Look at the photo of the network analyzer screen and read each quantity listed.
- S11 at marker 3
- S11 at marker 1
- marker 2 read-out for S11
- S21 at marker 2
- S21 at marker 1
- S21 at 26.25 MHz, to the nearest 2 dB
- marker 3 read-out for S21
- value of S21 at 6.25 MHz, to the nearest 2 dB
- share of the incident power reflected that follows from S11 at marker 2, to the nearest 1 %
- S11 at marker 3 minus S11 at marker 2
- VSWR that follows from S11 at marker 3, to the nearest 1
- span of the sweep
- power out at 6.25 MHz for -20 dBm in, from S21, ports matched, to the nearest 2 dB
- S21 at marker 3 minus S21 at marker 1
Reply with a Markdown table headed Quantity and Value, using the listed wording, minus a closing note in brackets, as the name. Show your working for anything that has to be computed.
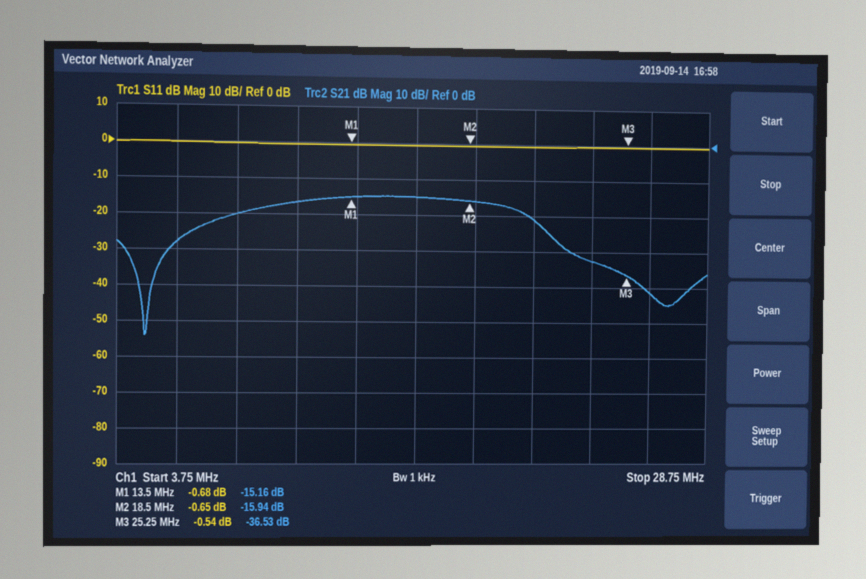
| Quantity | Value |
|---|---|
| S11 at marker 3 | -0.54 dB |
| S11 at marker 1 | -0.68 dB |
| marker 2 read-out for S11 | -0.65 dB |
| S21 at marker 2 | -15.94 dB |
| S21 at marker 1 | -15.16 dB |
| S21 at 26.25 MHz, to the nearest 2 dB | -42 dB |
| marker 3 read-out for S21 | -36.53 dB |
| value of S21 at 6.25 MHz, to the nearest 2 dB | -28 dB |
| share of the incident power reflected that follows from S11 at marker 2, to the nearest 1 % | 10^(-0.65/10) ≈ 86 % |
| S11 at marker 3 minus S11 at marker 2 | -0.54 − (-0.65) = 0.11 dB |
| VSWR that follows from S11 at marker 3, to the nearest 1 | (1 + 0.9397)/(1 − 0.9397) ≈ 32 |
| span of the sweep | 25 MHz |
| power out at 6.25 MHz for -20 dBm in, from S21, ports matched, to the nearest 2 dB | -20 dBm + (-28 dB) = -48 dBm |
| S21 at marker 3 minus S21 at marker 1 | -36.53 − (-15.16) = -21.37 dB |
